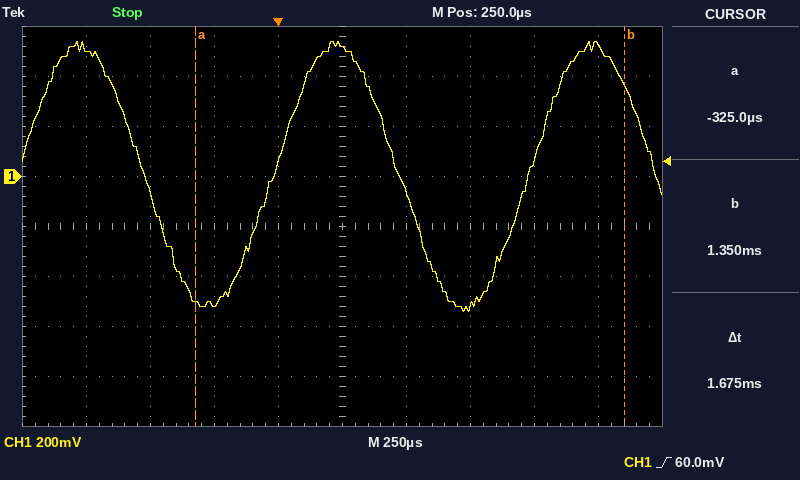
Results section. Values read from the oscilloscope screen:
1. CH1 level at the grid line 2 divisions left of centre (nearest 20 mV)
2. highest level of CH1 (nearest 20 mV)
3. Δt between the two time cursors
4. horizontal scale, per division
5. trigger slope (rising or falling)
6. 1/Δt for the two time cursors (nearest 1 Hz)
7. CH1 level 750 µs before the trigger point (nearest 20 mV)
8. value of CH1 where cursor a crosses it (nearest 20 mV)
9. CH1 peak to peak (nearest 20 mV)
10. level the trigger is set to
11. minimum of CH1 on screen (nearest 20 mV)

-520 mV
540 mV
1.675 ms
250 µs
rising
597 Hz
520 mV
-500 mV
1.08 V
60.0 mV
-540 mV
